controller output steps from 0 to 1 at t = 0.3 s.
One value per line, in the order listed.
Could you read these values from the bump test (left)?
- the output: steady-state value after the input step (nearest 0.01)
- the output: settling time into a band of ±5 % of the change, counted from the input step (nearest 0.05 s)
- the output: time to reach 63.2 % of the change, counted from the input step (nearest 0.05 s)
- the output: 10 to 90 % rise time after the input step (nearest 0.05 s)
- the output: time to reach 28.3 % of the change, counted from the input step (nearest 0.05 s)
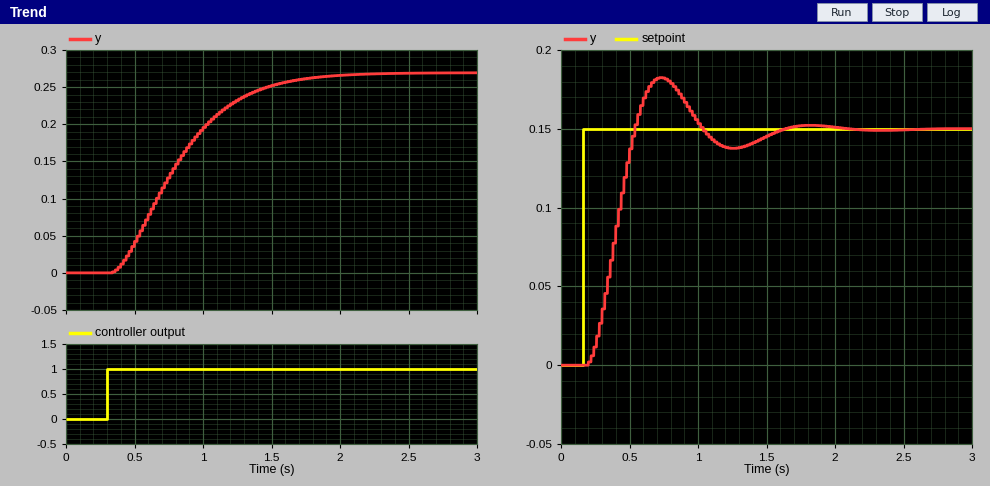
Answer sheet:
0.27
1.30 s
0.60 s
0.90 s
0.30 s
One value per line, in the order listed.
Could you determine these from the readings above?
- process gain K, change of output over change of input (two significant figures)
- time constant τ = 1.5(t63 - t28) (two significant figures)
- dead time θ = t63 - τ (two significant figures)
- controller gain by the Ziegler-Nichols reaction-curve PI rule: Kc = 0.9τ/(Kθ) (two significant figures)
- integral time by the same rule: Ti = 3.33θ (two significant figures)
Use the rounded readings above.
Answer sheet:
0.27
0.45 s
0.15 s
10
0.50 s
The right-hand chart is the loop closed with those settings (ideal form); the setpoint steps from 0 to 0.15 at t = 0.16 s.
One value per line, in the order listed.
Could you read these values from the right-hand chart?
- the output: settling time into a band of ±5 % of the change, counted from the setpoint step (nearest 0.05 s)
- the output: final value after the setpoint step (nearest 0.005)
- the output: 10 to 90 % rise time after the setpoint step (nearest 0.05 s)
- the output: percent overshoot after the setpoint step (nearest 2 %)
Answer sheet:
1.30 s
0.150
0.25 s
22 %
